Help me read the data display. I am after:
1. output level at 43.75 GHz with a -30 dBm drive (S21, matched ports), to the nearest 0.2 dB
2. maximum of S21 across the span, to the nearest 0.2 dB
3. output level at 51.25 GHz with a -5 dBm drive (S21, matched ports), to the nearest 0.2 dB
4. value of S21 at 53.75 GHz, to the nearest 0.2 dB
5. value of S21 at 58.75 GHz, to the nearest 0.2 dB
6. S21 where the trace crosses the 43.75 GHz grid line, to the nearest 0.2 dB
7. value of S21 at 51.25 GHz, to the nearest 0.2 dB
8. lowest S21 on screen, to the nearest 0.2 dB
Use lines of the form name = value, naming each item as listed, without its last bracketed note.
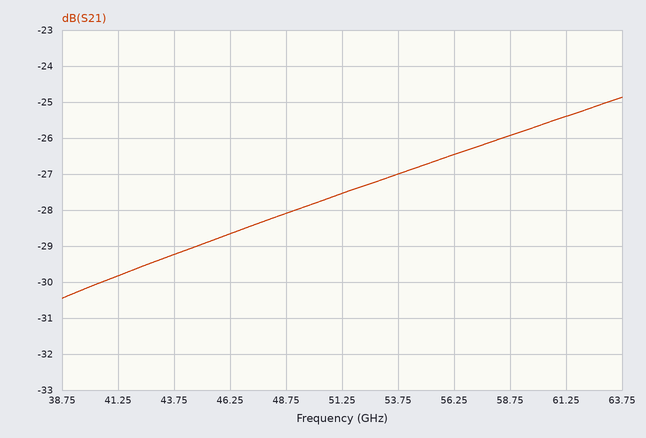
output level at 43.75 GHz with a -30 dBm drive (S21, matched ports), to the nearest 0.2 dB = -59.2 dBm
maximum of S21 across the span, to the nearest 0.2 dB = -24.8 dB
output level at 51.25 GHz with a -5 dBm drive (S21, matched ports), to the nearest 0.2 dB = -32.6 dBm
value of S21 at 53.75 GHz, to the nearest 0.2 dB = -27.0 dB
value of S21 at 58.75 GHz, to the nearest 0.2 dB = -26.0 dB
S21 where the trace crosses the 43.75 GHz grid line, to the nearest 0.2 dB = -29.2 dB
value of S21 at 51.25 GHz, to the nearest 0.2 dB = -27.6 dB
lowest S21 on screen, to the nearest 0.2 dB = -30.4 dB
